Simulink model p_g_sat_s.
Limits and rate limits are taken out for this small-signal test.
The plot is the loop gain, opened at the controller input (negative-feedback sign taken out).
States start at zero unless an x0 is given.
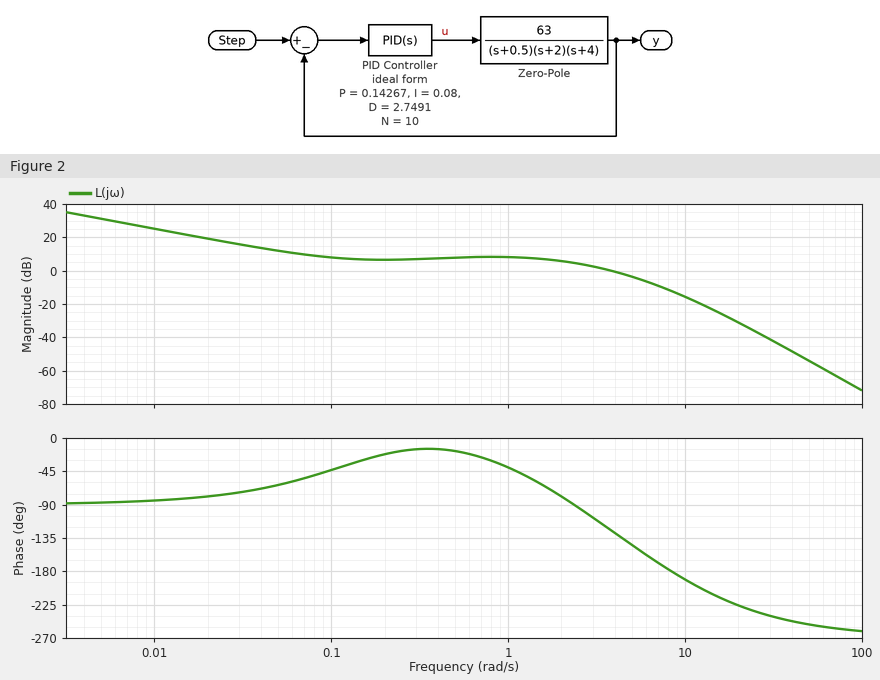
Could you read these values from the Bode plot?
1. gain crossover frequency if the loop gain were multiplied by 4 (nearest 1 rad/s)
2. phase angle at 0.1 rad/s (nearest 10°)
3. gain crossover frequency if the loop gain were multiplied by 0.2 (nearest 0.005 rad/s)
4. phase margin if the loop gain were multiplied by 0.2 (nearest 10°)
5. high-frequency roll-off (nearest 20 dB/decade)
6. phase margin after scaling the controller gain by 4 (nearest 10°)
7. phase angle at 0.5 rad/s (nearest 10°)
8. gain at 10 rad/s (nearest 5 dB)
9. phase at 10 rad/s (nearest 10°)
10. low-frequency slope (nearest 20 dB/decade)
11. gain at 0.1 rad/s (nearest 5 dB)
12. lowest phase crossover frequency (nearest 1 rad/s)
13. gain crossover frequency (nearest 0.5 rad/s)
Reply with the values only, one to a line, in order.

8 rad/s
-40°
0.040 rad/s
110°
-60 dB/decade
0°
-20°
-15 dB
-190°
-20 dB/decade
10 dB
8 rad/s
4.0 rad/s
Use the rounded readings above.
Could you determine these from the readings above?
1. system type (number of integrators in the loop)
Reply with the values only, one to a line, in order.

1
